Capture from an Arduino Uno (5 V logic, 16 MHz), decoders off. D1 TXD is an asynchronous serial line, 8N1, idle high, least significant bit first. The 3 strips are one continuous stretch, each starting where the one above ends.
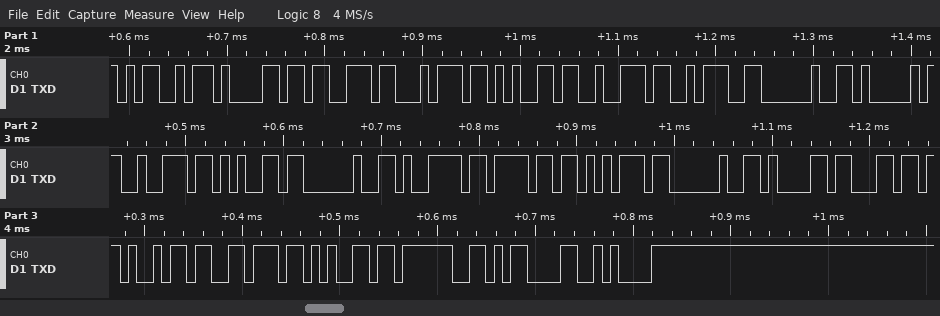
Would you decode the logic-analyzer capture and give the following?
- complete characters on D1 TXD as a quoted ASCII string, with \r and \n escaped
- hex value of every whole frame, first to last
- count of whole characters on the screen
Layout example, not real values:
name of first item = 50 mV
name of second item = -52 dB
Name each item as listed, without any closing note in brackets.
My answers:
complete characters on D1 TXD as a quoted ASCII string, with \r and \n escaped = "Master: Are you alive?\r\n"
hex value of every whole frame, first to last = 4D 61 73 74 65 72 3A 20 41 72 65 20 79 6F 75 20 61 6C 69 76 65 3F 0D 0A
count of whole characters on the screen = 24
